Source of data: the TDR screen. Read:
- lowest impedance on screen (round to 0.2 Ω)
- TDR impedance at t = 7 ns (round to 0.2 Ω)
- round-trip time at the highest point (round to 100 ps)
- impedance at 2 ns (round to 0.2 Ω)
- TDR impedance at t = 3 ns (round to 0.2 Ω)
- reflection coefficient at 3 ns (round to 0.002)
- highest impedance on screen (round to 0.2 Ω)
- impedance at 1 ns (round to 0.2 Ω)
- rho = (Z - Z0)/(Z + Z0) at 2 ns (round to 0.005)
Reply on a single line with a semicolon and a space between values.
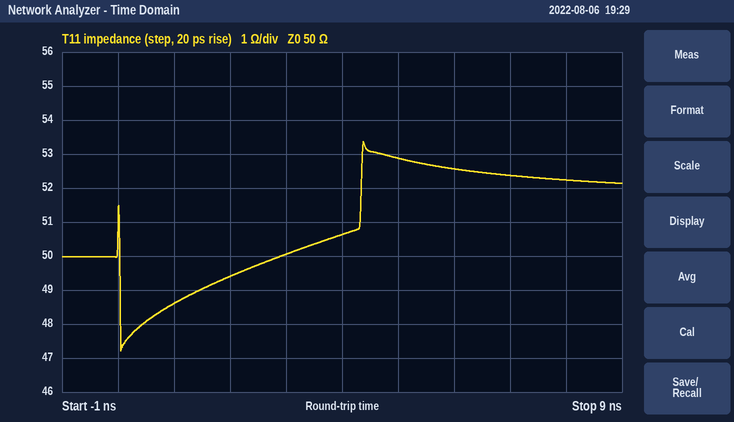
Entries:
47.2 Ω; 52.4 Ω; 4.4 ns; 49.4 Ω; 50.0 Ω; 0.000; 53.4 Ω; 48.6 Ω; -0.005
